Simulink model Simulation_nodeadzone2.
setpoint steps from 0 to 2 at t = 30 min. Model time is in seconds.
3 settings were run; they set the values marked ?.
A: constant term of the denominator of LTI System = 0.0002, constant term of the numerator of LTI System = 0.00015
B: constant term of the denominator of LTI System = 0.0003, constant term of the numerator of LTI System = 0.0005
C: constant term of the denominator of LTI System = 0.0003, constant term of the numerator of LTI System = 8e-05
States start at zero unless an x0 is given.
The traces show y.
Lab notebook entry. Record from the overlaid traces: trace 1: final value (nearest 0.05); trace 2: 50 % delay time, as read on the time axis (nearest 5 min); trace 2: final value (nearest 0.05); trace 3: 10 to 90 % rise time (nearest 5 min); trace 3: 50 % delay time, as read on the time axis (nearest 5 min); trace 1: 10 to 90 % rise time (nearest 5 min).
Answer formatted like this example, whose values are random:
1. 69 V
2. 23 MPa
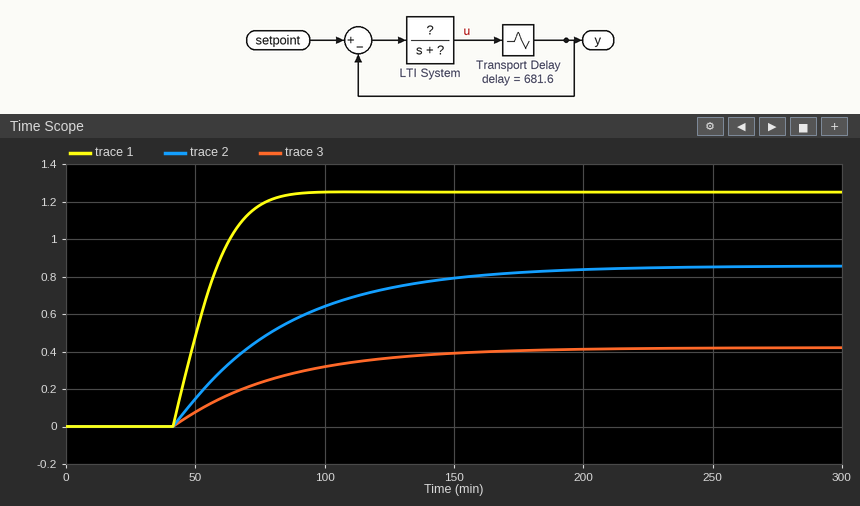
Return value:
1. 1.25
2. 70 min
3. 0.85
4. 90 min
5. 70 min
6. 25 min
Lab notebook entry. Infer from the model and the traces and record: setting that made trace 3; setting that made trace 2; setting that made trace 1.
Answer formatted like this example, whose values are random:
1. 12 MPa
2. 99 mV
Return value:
1. C
2. A
3. B
